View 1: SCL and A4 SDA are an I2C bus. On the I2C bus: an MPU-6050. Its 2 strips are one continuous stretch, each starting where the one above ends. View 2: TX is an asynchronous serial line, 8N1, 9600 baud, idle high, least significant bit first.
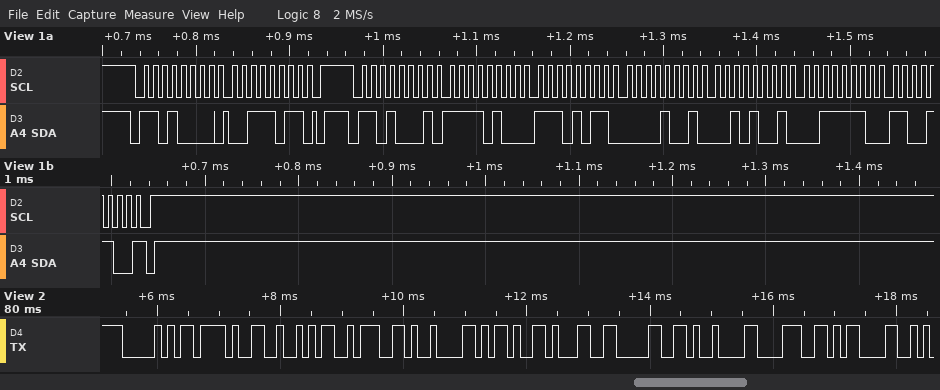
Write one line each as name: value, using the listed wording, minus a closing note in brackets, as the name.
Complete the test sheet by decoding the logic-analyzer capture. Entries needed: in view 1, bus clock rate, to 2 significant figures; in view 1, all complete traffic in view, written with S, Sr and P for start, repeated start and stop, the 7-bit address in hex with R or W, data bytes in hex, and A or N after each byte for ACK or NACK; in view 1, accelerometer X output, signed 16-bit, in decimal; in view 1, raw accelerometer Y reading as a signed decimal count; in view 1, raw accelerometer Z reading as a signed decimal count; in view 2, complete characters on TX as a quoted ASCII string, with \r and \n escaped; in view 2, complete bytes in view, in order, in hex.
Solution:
in view 1, bus clock rate, to 2 significant figures: 100 kHz
in view 1, all complete traffic in view, written with S, Sr and P for start, repeated start and stop, the 7-bit address in hex with R or W, data bytes in hex, and A or N after each byte for ACK or NACK: S 68W A 3B A P S 68R A F4 A EB A 09 A 29 A 3E A CC N P
in view 1, accelerometer X output, signed 16-bit, in decimal: -2837
in view 1, raw accelerometer Y reading as a signed decimal count: 2345
in view 1, raw accelerometer Z reading as a signed decimal count: 16076
in view 2, complete characters on TX as a quoted ASCII string, with \r and \n escaped: "P/R:\t-10\t8\r"
in view 2, complete bytes in view, in order, in hex: 50 2F 52 3A 09 2D 31 30 09 38 0D
